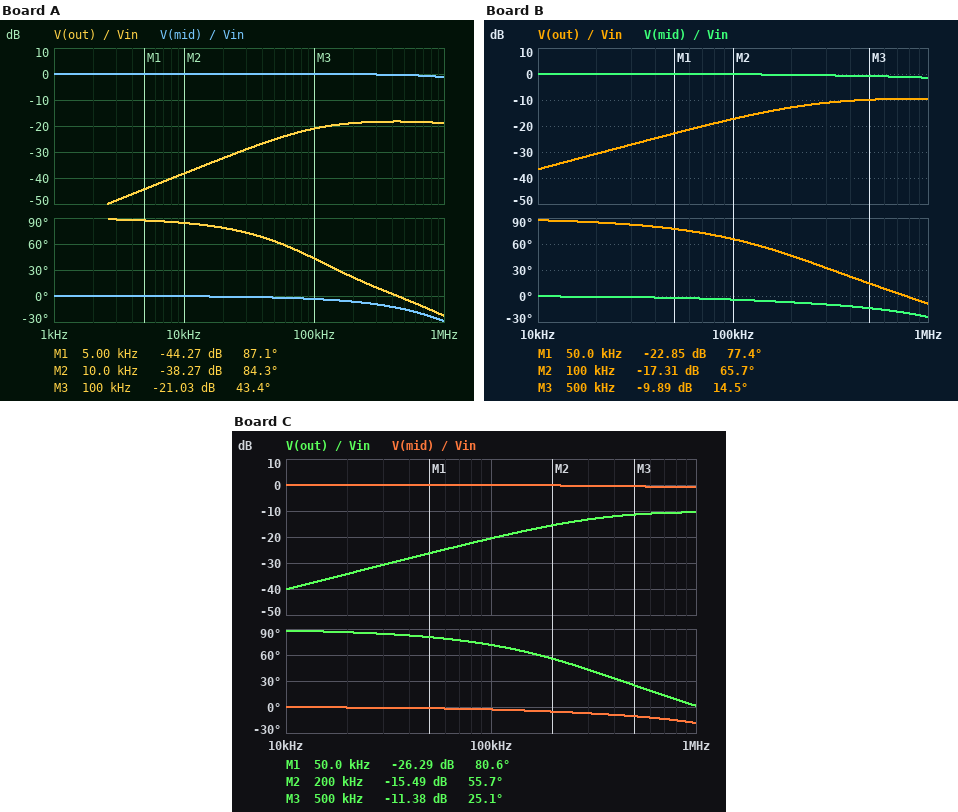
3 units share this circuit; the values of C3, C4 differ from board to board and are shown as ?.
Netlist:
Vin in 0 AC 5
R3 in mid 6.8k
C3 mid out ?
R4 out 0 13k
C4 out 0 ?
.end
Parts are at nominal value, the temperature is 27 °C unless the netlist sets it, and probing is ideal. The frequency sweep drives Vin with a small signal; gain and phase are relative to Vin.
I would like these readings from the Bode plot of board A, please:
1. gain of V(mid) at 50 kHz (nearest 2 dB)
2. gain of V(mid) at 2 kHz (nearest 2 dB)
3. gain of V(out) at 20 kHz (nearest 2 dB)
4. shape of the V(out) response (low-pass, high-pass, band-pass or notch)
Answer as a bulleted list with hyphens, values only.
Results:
- 0 dB
- 0 dB
- -32 dB
- high-pass
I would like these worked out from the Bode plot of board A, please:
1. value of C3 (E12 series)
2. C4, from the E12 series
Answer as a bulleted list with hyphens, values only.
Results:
- 15 pF
- 100 pF
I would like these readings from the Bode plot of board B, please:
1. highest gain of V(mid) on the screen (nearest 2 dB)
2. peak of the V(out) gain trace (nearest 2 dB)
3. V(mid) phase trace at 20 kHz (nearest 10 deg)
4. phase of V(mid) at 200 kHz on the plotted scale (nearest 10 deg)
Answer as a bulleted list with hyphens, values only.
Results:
- 0 dB
- -10 dB
- 0 deg
- -10 deg
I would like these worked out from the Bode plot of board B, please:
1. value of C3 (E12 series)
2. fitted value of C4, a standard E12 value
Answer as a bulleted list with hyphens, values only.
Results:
- 18 pF
- 27 pF
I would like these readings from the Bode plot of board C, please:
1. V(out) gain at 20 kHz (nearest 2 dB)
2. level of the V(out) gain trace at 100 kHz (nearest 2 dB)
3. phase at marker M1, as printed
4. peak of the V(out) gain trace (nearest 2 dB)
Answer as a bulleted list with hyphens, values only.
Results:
- -34 dB
- -20 dB
- 80.6 deg
- -10 dB
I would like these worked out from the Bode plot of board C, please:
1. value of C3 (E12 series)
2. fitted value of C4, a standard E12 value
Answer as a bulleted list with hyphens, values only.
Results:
- 12 pF
- 22 pF
